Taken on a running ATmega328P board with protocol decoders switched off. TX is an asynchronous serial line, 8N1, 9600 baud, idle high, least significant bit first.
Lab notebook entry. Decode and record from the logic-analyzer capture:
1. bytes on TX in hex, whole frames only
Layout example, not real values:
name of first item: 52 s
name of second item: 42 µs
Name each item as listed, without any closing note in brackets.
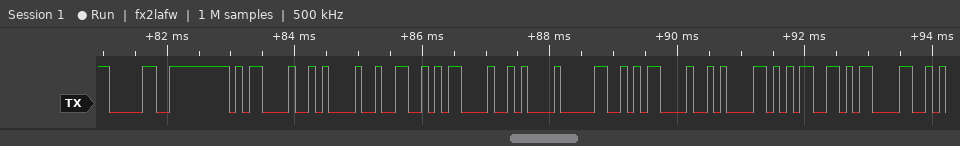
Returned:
bytes on TX in hex, whole frames only: 0x30 0x0D 0x0A 0x32 0x0D 0x0A 0x30 0x0D 0x0A 0x35 0x0D
